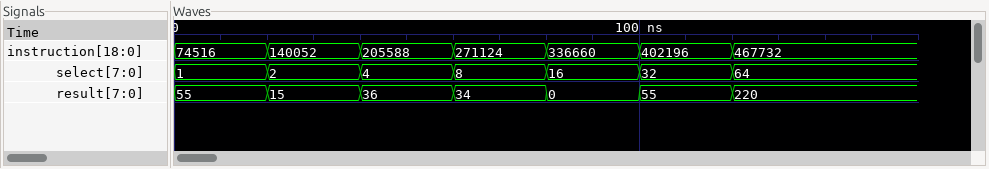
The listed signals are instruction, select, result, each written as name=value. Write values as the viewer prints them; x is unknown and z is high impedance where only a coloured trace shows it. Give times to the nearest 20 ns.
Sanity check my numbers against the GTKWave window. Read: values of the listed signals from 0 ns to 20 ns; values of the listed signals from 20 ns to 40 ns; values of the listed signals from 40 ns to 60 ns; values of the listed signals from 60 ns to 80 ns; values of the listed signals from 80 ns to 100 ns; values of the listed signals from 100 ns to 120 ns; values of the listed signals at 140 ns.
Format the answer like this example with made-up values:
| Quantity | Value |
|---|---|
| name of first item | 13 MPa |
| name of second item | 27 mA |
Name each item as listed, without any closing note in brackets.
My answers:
| Quantity | Value |
|---|---|
| values of the listed signals from 0 ns to 20 ns | instruction=74516, select=1, result=55 |
| values of the listed signals from 20 ns to 40 ns | instruction=140052, select=2, result=15 |
| values of the listed signals from 40 ns to 60 ns | instruction=205588, select=4, result=36 |
| values of the listed signals from 60 ns to 80 ns | instruction=271124, select=8, result=34 |
| values of the listed signals from 80 ns to 100 ns | instruction=336660, select=16, result=0 |
| values of the listed signals from 100 ns to 120 ns | instruction=402196, select=32, result=55 |
| values of the listed signals at 140 ns | instruction=467732, select=64, result=220 |
